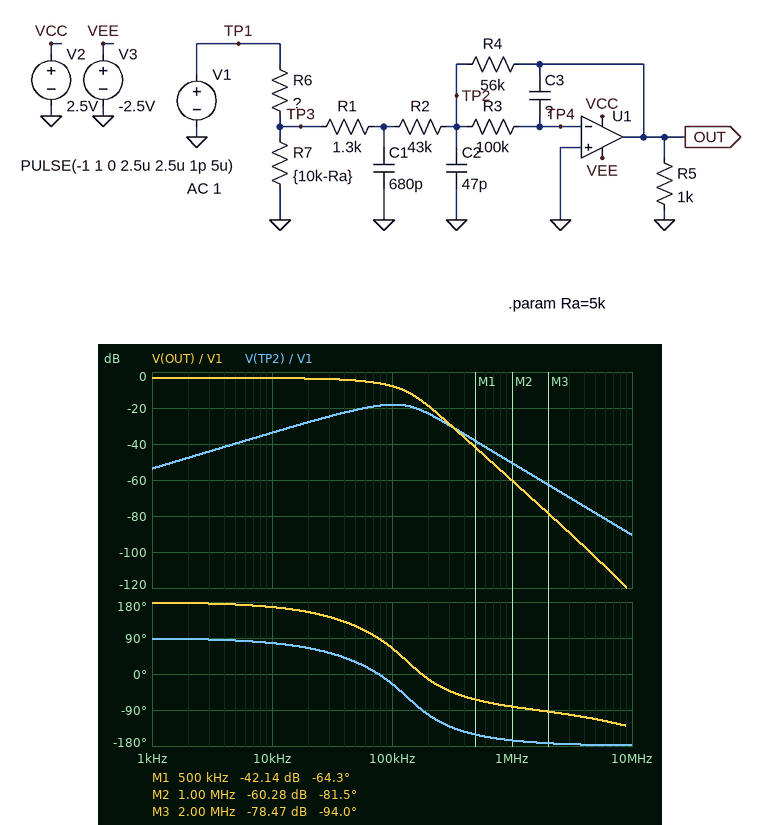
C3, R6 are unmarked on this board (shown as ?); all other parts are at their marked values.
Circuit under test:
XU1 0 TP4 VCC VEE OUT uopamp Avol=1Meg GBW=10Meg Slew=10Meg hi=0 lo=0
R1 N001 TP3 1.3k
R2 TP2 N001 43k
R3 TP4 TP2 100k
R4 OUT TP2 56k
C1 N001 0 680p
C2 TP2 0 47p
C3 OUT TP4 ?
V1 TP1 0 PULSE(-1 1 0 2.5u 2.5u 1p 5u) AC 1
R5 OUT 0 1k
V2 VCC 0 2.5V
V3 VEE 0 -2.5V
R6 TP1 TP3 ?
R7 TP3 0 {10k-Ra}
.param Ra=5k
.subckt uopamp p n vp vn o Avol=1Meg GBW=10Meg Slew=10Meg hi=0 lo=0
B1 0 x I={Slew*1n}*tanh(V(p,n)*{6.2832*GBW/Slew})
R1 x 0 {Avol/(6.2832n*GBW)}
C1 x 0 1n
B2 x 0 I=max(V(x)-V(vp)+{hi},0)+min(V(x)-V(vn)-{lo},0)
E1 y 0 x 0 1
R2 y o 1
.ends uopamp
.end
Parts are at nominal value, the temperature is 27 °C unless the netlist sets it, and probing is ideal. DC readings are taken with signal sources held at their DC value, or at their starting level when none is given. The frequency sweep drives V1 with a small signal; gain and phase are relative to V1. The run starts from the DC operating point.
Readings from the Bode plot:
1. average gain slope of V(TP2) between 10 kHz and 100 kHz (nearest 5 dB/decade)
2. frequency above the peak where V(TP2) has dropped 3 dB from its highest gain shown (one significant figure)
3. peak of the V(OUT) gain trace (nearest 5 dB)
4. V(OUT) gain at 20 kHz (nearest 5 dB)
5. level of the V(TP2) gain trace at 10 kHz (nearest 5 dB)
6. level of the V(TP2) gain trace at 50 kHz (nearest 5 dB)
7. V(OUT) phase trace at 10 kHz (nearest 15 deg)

15 dB/decade
200 kHz
-5 dB
-5 dB
-35 dB
-20 dB
165 deg
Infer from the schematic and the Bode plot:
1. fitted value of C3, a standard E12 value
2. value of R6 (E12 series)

4.7 pF
3.9 kΩ
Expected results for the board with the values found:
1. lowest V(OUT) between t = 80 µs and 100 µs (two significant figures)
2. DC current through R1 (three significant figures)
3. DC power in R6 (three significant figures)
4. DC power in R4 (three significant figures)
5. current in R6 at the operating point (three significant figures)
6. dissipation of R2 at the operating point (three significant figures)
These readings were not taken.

-94 mV
12.1 µA
55.4 µW
8.18 µW
119 µA
6.28 µW
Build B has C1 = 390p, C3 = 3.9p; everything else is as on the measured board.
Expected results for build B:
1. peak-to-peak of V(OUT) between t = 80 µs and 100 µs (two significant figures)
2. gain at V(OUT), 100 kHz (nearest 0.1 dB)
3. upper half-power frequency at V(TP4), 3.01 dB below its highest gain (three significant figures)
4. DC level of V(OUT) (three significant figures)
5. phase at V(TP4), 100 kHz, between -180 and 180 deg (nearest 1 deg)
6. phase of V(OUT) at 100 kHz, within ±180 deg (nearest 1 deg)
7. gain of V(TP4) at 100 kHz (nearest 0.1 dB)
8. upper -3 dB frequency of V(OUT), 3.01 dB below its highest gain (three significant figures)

370 mV
-4.6 dB
200 kHz
677 mV
0 deg
90 deg
-44.6 dB
134 kHz
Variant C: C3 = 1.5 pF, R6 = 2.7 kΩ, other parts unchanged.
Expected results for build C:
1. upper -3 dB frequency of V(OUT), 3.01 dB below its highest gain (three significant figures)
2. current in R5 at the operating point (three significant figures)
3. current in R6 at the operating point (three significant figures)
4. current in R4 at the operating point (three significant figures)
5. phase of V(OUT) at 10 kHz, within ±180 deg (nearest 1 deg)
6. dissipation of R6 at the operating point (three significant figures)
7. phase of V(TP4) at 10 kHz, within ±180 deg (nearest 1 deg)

110 kHz
790 µA
139 µA
14.1 µA
171 deg
52.2 µW
81 deg
